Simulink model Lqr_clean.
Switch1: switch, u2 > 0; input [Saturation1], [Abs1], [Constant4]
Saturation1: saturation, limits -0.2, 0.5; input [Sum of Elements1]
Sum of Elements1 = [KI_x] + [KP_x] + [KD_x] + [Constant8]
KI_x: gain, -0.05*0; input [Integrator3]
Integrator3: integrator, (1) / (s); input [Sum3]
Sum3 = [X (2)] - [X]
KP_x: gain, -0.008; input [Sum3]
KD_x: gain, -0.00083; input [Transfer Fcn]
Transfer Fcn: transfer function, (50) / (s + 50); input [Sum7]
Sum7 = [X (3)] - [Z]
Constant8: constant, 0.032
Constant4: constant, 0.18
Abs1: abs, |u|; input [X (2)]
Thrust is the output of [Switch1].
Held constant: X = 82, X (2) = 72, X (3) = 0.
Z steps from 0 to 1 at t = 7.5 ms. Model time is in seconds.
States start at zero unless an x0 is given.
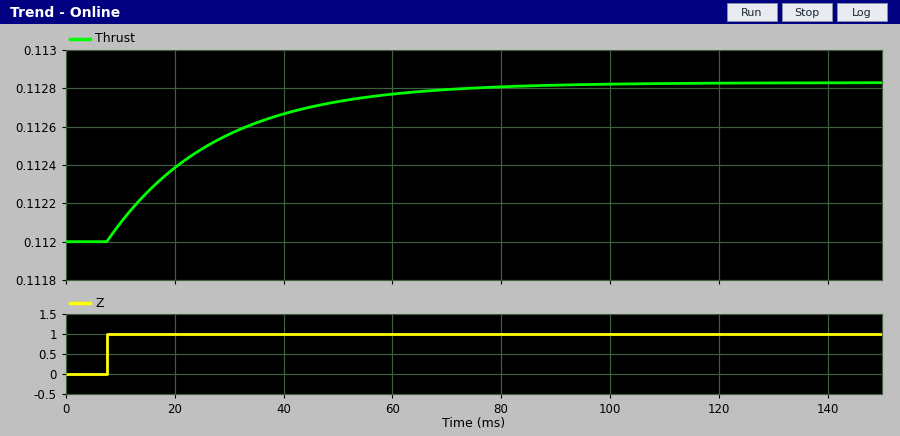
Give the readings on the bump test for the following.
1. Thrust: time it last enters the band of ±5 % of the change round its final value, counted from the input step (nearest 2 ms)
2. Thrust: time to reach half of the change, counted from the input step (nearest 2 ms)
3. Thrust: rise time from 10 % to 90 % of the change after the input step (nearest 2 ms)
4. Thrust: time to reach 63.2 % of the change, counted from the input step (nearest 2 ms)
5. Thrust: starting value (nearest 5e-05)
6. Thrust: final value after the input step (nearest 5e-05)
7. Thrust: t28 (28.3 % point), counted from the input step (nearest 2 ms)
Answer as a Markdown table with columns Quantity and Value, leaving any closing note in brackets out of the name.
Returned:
| Quantity | Value |
|---|---|
| Thrust: time it last enters the band of ±5 % of the change round its final value, counted from the input step | 60 ms |
| Thrust: time to reach half of the change, counted from the input step | 14 ms |
| Thrust: rise time from 10 % to 90 % of the change after the input step | 44 ms |
| Thrust: time to reach 63.2 % of the change, counted from the input step | 20 ms |
| Thrust: starting value | 0.11200 |
| Thrust: final value after the input step | 0.11285 |
| Thrust: t28 (28.3 % point), counted from the input step | 6 ms |
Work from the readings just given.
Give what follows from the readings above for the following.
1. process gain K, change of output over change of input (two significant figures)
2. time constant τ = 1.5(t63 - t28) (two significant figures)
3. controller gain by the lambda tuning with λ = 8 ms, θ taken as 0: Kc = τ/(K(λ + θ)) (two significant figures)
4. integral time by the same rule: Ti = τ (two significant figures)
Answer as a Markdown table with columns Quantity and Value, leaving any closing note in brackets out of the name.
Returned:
| Quantity | Value |
|---|---|
| process gain K, change of output over change of input | 0.00085 |
| time constant τ = 1.5(t63 - t28) | 21 ms |
| controller gain by the lambda tuning with λ = 8 ms, θ taken as 0: Kc = τ/(K(λ + θ)) | 3100 |
| integral time by the same rule: Ti = τ | 21 ms |
